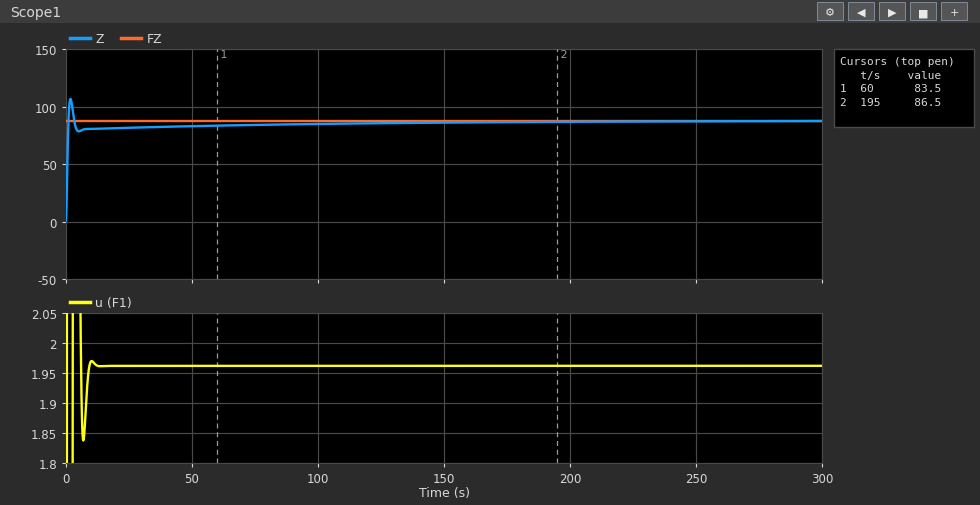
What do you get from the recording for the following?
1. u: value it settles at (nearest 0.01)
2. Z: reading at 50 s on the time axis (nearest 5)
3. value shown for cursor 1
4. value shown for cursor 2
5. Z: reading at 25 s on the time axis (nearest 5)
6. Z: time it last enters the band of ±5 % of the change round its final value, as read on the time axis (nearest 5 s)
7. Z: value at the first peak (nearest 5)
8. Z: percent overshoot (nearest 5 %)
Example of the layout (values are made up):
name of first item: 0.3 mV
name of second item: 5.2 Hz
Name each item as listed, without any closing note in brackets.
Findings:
u: value it settles at: 1.96
Z: reading at 50 s on the time axis: 85
value shown for cursor 1: 83.5
value shown for cursor 2: 86.5
Z: reading at 25 s on the time axis: 80
Z: time it last enters the band of ±5 % of the change round its final value, as read on the time axis: 60 s
Z: value at the first peak: 105
Z: percent overshoot: 20 %
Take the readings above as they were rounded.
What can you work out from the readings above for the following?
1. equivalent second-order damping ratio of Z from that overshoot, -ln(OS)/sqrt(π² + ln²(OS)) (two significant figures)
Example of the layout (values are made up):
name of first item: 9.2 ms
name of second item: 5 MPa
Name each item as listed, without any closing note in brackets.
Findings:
equivalent second-order damping ratio of Z from that overshoot, -ln(OS)/sqrt(π² + ln²(OS)): 0.46
